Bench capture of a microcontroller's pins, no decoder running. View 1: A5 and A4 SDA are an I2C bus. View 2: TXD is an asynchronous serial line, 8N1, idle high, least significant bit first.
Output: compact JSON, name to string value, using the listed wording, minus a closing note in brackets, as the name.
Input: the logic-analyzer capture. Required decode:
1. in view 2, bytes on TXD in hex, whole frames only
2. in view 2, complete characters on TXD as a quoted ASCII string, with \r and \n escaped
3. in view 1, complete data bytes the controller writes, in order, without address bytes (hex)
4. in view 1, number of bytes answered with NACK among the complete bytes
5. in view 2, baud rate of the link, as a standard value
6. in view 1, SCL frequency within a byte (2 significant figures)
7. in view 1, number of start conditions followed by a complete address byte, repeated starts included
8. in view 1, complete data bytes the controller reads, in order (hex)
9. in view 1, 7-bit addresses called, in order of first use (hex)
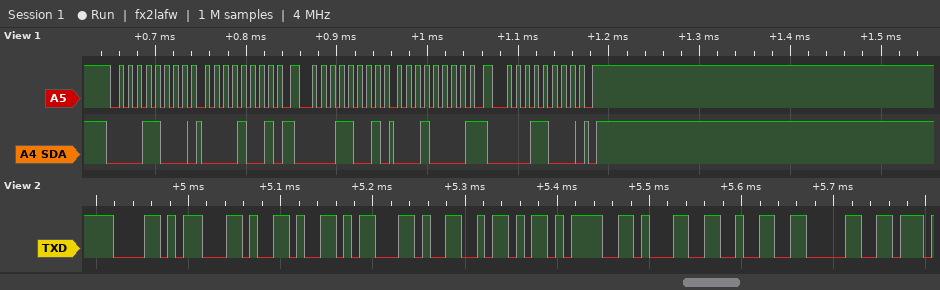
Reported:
{"in view 2, bytes on TXD in hex, whole frames only": "58 2C 59 2C 5A 3D 31 32 30", "in view 2, complete characters on TXD as a quoted ASCII string, with \\r and \\n escaped": "\"X,Y,Z=120\"", "in view 1, complete data bytes the controller writes, in order, without address bytes": "09", "in view 1, number of bytes answered with NACK among the complete bytes": "1", "in view 2, baud rate of the link, as a standard value": "115200 baud", "in view 1, SCL frequency within a byte": "100 kHz", "in view 1, number of start conditions followed by a complete address byte, repeated starts included": "3", "in view 1, complete data bytes the controller reads, in order": "10", "in view 1, 7-bit addresses called, in order of first use": "0x0C"}
